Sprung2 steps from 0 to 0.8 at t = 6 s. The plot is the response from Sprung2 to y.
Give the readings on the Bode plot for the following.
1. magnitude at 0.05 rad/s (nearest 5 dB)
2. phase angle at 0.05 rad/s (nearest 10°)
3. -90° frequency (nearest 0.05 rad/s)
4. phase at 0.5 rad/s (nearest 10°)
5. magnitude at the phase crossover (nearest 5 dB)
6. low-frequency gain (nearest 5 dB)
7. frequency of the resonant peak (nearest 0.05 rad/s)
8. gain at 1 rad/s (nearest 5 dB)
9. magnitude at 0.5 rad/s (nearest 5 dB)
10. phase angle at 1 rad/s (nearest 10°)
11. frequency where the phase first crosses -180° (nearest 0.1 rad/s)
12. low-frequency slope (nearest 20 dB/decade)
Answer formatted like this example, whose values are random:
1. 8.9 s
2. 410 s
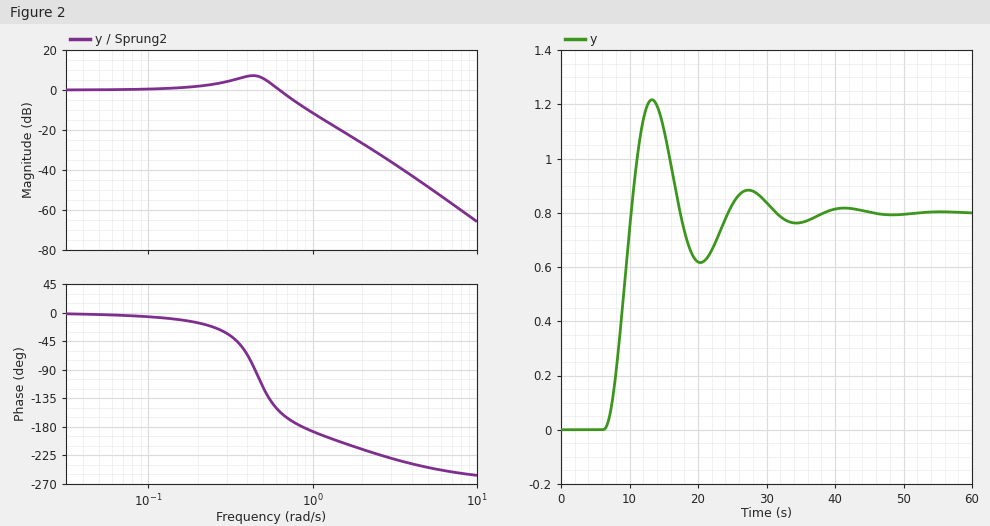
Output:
1. 0 dB
2. 0°
3. 0.45 rad/s
4. -120°
5. -10 dB
6. 0 dB
7. 0.45 rad/s
8. -10 dB
9. 5 dB
10. -190°
11. 0.9 rad/s
12. 0 dB/decade
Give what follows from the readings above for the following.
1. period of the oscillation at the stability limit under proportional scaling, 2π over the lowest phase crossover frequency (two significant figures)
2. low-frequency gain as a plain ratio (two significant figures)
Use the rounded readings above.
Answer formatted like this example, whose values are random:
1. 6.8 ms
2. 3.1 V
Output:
1. 7.0 s
2. 1.0
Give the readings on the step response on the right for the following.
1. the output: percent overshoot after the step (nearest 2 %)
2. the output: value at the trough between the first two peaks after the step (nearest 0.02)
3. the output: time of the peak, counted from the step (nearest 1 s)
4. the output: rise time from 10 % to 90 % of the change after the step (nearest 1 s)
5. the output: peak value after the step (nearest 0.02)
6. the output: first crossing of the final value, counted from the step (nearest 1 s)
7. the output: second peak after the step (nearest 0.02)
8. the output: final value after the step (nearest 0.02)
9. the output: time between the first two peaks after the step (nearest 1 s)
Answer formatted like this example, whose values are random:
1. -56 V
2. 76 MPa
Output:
1. 52 %
2. 0.62
3. 7 s
4. 3 s
5. 1.22
6. 4 s
7. 0.88
8. 0.80
9. 14 s
